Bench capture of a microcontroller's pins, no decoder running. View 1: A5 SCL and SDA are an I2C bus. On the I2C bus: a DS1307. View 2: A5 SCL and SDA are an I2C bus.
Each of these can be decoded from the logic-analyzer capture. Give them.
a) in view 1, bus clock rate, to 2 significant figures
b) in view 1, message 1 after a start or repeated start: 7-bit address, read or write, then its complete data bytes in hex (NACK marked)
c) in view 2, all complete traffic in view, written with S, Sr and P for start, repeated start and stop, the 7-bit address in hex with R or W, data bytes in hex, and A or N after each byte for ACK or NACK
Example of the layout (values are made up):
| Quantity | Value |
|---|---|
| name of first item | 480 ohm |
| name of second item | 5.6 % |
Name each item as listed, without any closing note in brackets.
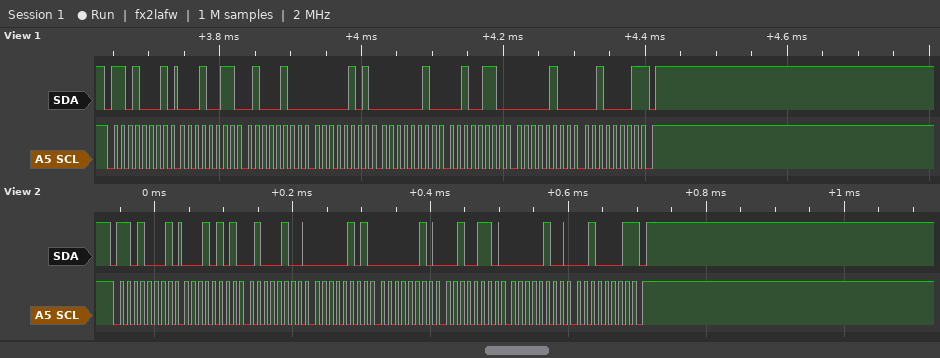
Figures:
| Quantity | Value |
|---|---|
| in view 1, bus clock rate, to 2 significant figures | 100 kHz |
| in view 1, message 1 after a start or repeated start: 7-bit address, read or write, then its complete data bytes in hex | 0x68 read: 13 44 05 02 26 04 21 NACK |
| in view 2, all complete traffic in view, written with S, Sr and P for start, repeated start and stop, the 7-bit address in hex with R or W, data bytes in hex, and A or N after each byte for ACK or NACK | S 68R A 15 A 44 A 05 A 02 A 26 A 04 A 21 N P |
